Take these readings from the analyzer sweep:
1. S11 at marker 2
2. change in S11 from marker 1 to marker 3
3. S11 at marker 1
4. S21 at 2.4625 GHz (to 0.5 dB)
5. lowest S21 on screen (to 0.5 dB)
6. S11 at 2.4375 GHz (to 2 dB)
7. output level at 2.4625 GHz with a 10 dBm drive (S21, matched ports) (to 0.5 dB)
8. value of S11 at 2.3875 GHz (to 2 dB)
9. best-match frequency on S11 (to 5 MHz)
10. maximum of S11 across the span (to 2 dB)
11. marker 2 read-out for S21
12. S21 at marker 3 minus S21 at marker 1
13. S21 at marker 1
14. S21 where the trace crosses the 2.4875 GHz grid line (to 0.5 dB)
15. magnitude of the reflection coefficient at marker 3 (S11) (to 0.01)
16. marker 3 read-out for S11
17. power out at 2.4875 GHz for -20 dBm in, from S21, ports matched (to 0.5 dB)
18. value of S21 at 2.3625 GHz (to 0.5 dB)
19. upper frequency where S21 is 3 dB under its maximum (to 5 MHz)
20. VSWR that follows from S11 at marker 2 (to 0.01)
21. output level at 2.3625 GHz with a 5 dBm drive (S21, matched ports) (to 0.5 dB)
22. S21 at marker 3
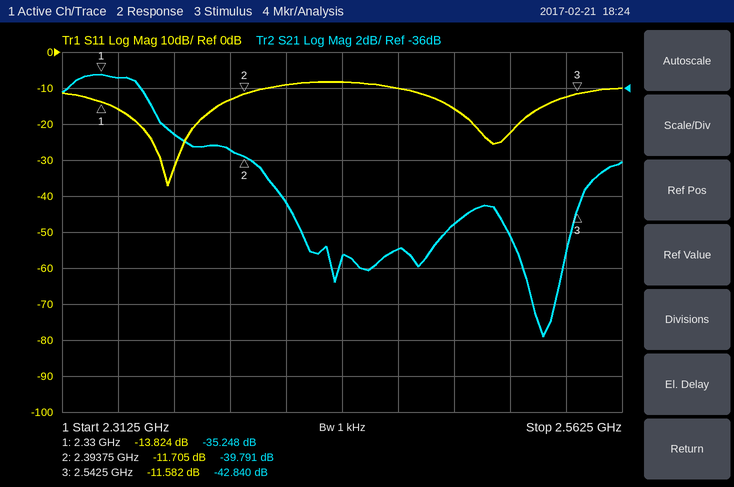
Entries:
-11.705 dB
2.242 dB
-13.824 dB
-45.0 dB
-50.0 dB
-8 dB
-35.0 dBm
-14 dB
2.360 GHz
-8 dB
-39.791 dB
-7.592 dB
-35.248 dB
-43.5 dB
0.26
-11.582 dB
-63.5 dBm
-38.5 dB
2.360 GHz
1.70
-33.5 dBm
-42.840 dB
